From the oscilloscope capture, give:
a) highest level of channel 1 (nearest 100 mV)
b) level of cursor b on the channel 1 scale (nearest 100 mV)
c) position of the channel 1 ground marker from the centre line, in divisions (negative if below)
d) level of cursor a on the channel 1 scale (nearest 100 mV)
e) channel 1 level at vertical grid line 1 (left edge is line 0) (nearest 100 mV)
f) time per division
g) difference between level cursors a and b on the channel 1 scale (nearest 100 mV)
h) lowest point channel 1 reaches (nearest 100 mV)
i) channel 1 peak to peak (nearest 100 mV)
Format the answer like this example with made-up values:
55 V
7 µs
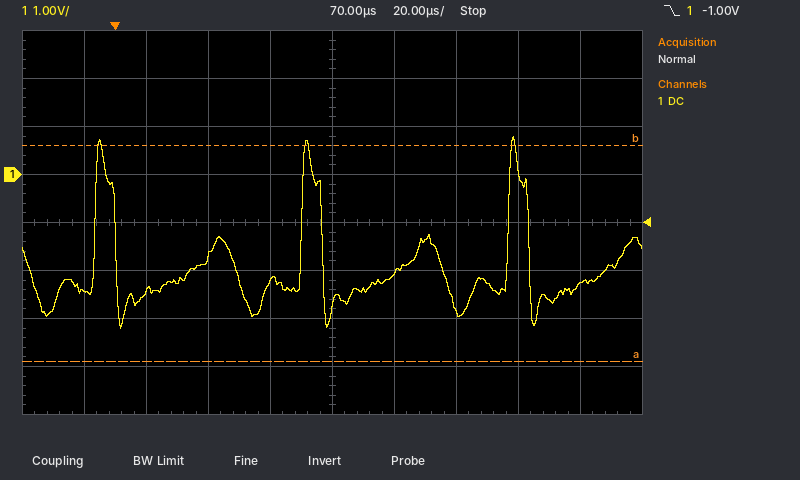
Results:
800 mV
600 mV
+1.0 div
-3.9 V
-2.4 V
20 µs
4.5 V
-3.2 V
4.0 V
